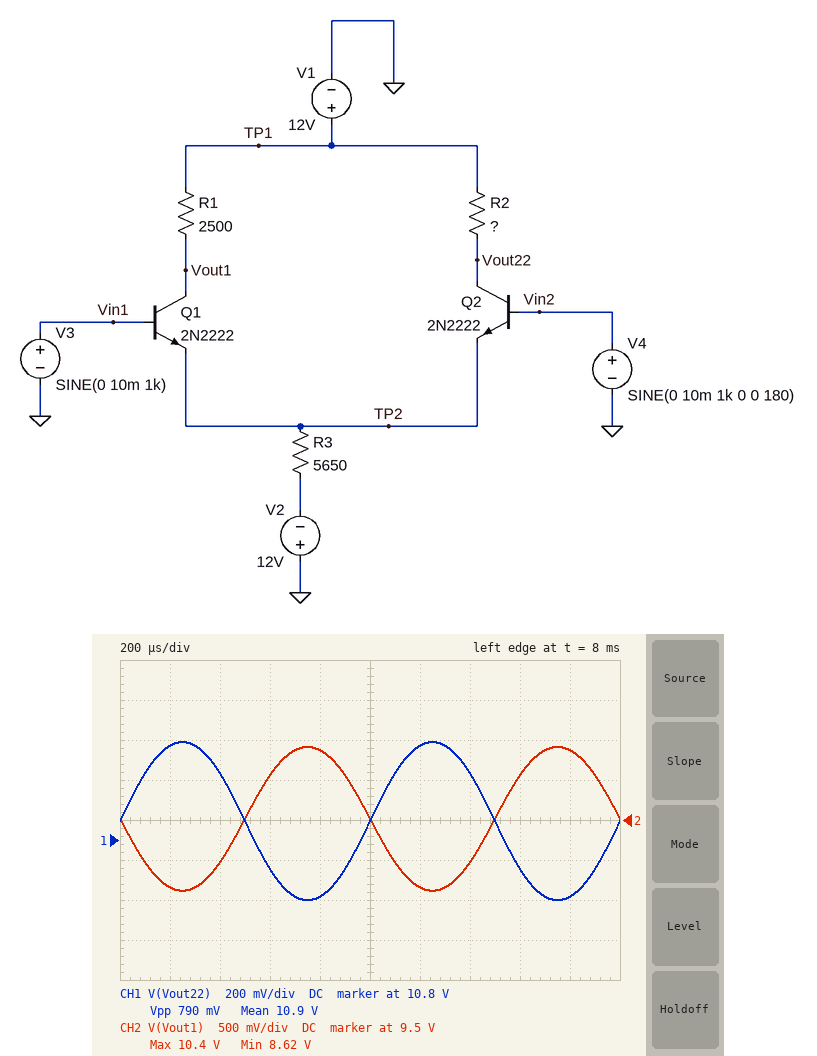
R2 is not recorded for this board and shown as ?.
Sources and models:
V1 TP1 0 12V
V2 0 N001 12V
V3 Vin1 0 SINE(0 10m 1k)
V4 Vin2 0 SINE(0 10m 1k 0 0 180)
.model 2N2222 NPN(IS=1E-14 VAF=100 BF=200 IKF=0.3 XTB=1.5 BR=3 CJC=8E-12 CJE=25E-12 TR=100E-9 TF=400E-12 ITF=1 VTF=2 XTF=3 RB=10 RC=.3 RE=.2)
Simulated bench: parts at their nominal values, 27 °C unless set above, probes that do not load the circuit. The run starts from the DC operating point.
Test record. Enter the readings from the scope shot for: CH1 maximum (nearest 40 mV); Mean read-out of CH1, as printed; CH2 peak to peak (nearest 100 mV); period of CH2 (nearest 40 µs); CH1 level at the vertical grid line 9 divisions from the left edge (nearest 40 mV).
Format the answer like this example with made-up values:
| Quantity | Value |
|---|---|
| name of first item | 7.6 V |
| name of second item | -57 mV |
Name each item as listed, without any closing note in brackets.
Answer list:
| Quantity | Value |
|---|---|
| CH1 maximum | 11.28 V |
| Mean read-out of CH1, as printed | 10.9 V |
| CH2 peak to peak | 1.8 V |
| period of CH2 | 1.00 ms |
| CH1 level at the vertical grid line 9 divisions from the left edge | 10.52 V |
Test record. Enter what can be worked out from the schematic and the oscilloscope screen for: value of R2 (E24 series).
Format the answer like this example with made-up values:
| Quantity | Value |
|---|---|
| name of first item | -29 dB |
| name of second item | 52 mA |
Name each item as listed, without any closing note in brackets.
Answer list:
| Quantity | Value |
|---|---|
| value of R2 | 1.1 kΩ |
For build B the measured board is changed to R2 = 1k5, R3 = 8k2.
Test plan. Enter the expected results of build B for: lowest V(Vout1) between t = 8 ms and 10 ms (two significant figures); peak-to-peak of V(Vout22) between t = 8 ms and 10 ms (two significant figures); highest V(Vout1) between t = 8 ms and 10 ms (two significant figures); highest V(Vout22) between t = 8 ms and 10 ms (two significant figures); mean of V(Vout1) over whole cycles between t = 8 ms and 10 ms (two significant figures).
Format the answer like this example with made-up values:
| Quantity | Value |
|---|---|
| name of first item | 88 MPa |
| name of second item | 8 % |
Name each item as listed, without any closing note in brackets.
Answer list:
| Quantity | Value |
|---|---|
| lowest V(Vout1) between t = 8 ms and 10 ms | 9.7 V |
| peak-to-peak of V(Vout22) between t = 8 ms and 10 ms | 750 mV |
| highest V(Vout1) between t = 8 ms and 10 ms | 11 V |
| highest V(Vout22) between t = 8 ms and 10 ms | 11 V |
| mean of V(Vout1) over whole cycles between t = 8 ms and 10 ms | 10 V |
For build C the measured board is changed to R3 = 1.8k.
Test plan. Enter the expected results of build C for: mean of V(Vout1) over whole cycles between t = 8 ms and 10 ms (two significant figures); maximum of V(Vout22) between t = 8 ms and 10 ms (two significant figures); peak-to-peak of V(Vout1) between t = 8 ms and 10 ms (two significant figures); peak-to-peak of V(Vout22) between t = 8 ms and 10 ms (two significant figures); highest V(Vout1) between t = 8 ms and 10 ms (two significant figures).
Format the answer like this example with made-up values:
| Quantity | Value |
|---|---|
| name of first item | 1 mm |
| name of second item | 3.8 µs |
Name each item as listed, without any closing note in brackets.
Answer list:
| Quantity | Value |
|---|---|
| mean of V(Vout1) over whole cycles between t = 8 ms and 10 ms | 4.3 V |
| maximum of V(Vout22) between t = 8 ms and 10 ms | 9.7 V |
| peak-to-peak of V(Vout1) between t = 8 ms and 10 ms | 5.3 V |
| peak-to-peak of V(Vout22) between t = 8 ms and 10 ms | 2.3 V |
| highest V(Vout1) between t = 8 ms and 10 ms | 7.0 V |
